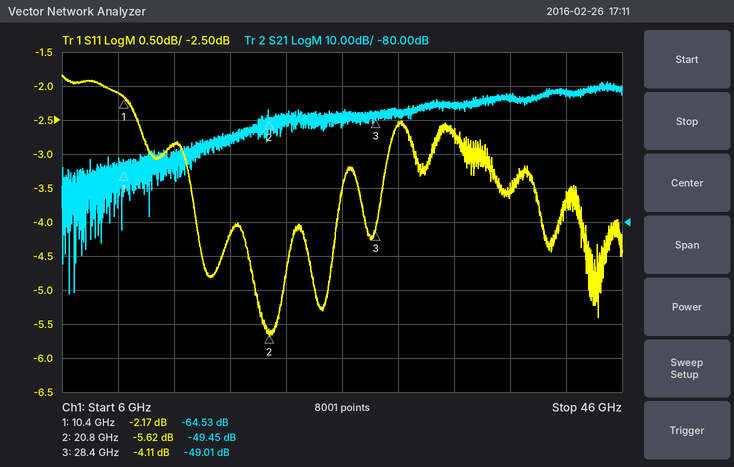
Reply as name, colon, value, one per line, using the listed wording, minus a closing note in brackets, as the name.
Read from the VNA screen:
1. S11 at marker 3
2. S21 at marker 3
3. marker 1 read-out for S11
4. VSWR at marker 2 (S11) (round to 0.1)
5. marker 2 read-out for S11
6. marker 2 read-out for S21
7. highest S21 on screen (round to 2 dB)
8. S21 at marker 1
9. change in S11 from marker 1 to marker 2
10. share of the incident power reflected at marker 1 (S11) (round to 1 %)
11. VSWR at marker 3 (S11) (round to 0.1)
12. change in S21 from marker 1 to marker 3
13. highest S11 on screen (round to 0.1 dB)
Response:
S11 at marker 3: -4.11 dB
S21 at marker 3: -49.01 dB
marker 1 read-out for S11: -2.17 dB
VSWR at marker 2 (S11): 3.2
marker 2 read-out for S11: -5.62 dB
marker 2 read-out for S21: -49.45 dB
highest S21 on screen: -38 dB
S21 at marker 1: -64.53 dB
change in S11 from marker 1 to marker 2: -3.45 dB
share of the incident power reflected at marker 1 (S11): 61 %
VSWR at marker 3 (S11): 4.3
change in S21 from marker 1 to marker 3: 15.52 dB
highest S11 on screen: -1.8 dB
